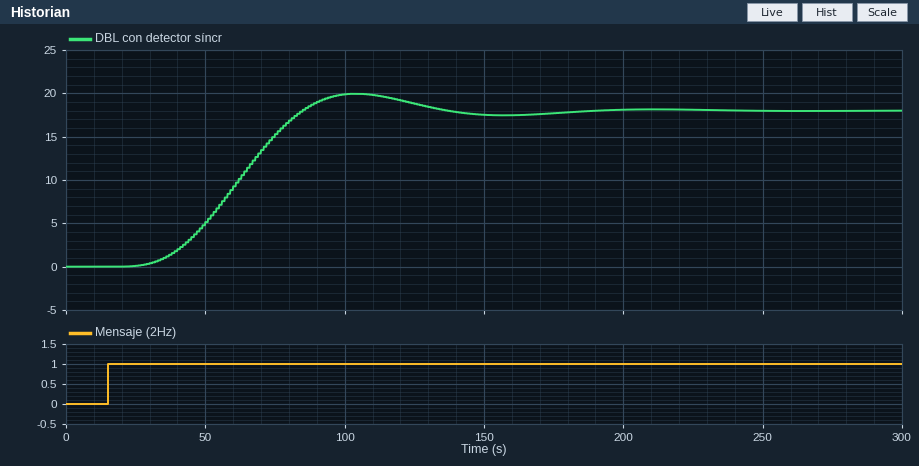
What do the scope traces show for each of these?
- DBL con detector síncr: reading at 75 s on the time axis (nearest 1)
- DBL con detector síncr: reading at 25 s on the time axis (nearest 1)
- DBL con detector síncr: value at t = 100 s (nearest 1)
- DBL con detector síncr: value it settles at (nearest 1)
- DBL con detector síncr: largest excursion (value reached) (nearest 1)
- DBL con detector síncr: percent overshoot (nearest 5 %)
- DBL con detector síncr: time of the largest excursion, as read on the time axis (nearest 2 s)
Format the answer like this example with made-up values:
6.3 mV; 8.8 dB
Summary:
15; 0; 20; 18; 20; 10 %; 104 s
